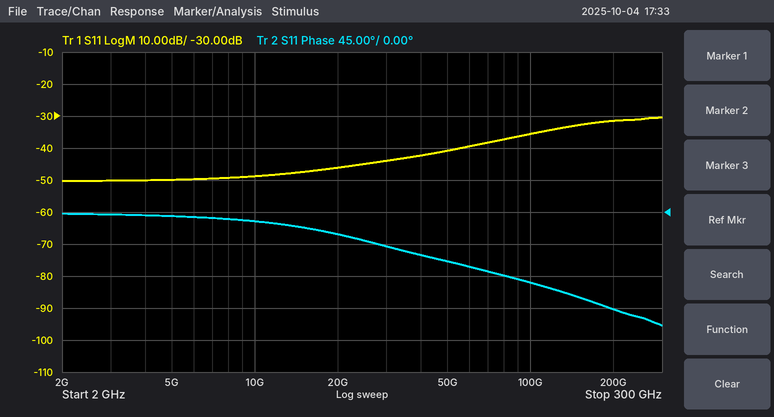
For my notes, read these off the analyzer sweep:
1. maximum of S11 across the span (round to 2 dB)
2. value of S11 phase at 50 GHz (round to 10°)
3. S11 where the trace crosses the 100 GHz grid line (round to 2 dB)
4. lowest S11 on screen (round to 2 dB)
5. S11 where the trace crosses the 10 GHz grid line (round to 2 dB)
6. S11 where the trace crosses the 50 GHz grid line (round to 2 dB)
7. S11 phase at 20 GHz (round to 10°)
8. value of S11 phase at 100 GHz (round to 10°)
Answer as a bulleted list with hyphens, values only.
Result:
- -30 dB
- -70°
- -36 dB
- -50 dB
- -48 dB
- -40 dB
- -30°
- -100°
